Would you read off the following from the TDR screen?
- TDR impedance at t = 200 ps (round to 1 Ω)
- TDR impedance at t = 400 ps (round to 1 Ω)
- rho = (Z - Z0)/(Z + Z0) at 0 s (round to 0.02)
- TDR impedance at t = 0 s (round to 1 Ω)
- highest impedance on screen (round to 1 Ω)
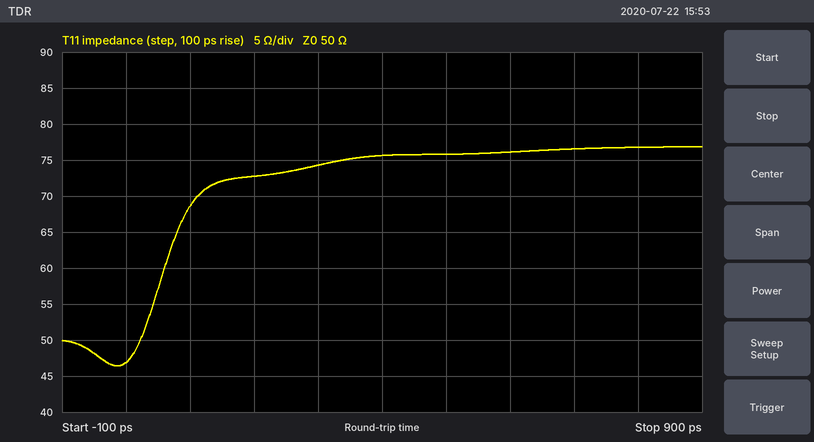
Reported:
73 Ω
76 Ω
-0.04
47 Ω
77 Ω
